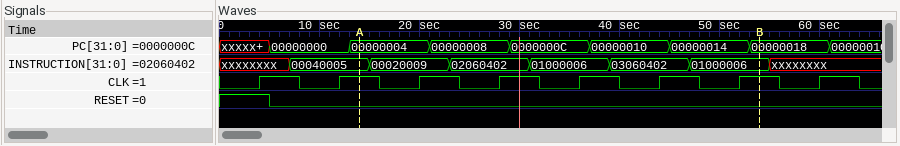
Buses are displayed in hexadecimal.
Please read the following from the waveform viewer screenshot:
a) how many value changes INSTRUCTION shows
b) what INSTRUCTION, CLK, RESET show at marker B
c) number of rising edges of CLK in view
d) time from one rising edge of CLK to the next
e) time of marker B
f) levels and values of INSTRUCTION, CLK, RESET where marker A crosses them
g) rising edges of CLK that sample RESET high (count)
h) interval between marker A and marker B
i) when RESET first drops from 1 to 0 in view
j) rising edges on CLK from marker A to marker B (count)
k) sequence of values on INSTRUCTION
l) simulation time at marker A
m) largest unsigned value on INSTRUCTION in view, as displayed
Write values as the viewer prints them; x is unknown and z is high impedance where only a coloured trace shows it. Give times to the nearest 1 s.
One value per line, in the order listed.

7
INSTRUCTION=01000006, CLK=1, RESET=0
8
8 s
54 s
INSTRUCTION=00040005, CLK=1, RESET=0
1
40 s
5 s
5
xxxxxxxx, 00040005, 00020009, 02060402, 01000006, 03060402, 01000006, xxxxxxxx
14 s
03060402
